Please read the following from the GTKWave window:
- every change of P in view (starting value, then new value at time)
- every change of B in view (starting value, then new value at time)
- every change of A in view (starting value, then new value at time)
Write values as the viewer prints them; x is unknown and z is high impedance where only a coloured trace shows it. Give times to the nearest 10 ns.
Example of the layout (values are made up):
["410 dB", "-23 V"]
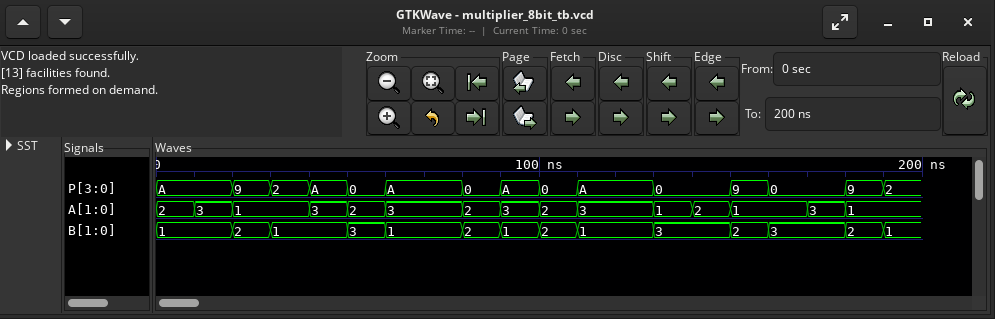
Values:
["A, 9 at 20 ns, 2 at 30 ns, A at 40 ns, 0 at 50 ns, A at 60 ns, 0 at 80 ns, A at 90 ns, 0 at 100 ns, A at 110 ns, 0 at 130 ns, 9 at 150 ns, 0 at 160 ns, 9 at 180 ns, 2 at 190 ns", "1, 2 at 20 ns, 1 at 30 ns, 3 at 50 ns, 1 at 60 ns, 2 at 80 ns, 1 at 90 ns, 2 at 100 ns, 1 at 110 ns, 3 at 130 ns, 2 at 150 ns, 3 at 160 ns, 2 at 180 ns, 1 at 190 ns", "2, 3 at 10 ns, 1 at 20 ns, 3 at 40 ns, 2 at 50 ns, 3 at 60 ns, 2 at 80 ns, 3 at 90 ns, 2 at 100 ns, 3 at 110 ns, 1 at 130 ns, 2 at 140 ns, 1 at 150 ns, 3 at 170 ns, 1 at 180 ns"]
